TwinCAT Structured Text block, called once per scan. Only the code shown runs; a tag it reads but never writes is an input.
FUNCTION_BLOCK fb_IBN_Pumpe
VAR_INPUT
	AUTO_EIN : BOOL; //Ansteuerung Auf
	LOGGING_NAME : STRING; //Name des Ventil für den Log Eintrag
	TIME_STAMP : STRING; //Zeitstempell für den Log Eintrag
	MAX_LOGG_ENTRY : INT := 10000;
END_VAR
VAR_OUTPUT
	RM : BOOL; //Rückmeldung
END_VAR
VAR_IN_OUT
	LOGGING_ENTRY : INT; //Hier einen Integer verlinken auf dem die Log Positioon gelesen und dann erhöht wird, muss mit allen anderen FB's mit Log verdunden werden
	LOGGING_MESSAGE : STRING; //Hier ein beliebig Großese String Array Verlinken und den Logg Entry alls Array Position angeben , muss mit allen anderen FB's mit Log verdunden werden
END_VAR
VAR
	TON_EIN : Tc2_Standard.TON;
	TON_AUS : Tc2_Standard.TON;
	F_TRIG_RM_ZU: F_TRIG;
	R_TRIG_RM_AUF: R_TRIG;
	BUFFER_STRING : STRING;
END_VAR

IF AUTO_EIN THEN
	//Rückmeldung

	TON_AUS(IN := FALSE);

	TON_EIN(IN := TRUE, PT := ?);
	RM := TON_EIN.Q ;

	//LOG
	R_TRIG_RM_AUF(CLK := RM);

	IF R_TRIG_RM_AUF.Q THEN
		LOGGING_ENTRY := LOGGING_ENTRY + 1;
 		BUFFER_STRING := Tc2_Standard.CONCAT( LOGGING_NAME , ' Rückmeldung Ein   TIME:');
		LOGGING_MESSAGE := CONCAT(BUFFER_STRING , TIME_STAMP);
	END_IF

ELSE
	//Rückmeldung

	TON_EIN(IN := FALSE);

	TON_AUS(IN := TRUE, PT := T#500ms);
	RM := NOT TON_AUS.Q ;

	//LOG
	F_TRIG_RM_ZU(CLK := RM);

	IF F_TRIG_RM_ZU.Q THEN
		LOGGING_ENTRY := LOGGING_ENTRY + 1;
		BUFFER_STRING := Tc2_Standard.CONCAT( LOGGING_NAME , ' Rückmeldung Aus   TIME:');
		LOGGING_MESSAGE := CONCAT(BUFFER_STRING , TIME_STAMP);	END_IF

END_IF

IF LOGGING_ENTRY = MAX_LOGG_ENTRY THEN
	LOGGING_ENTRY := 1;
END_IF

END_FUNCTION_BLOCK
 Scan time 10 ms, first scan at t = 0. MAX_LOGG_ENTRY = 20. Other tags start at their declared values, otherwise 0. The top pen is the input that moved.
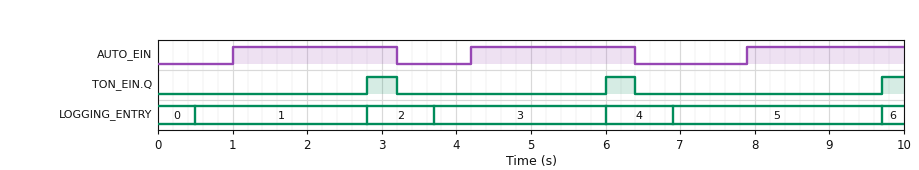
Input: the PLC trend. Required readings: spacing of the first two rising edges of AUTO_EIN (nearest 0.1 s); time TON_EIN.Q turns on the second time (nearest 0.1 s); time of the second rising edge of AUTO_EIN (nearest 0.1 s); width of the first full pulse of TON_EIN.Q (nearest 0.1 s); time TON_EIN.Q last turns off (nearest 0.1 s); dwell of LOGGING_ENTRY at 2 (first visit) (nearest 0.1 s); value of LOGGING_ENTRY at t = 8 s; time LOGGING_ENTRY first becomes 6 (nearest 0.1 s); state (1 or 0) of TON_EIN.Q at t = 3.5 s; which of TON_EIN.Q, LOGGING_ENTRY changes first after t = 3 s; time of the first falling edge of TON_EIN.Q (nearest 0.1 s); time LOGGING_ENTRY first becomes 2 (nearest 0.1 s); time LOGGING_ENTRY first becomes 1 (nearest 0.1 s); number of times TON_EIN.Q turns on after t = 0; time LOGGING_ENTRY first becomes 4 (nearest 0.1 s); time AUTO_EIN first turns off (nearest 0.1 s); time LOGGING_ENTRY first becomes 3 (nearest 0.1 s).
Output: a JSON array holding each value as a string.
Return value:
["3.2 s", "6.0 s", "4.2 s", "0.4 s", "6.4 s", "0.9 s", "5", "9.7 s", "0", "TON_EIN.Q", "3.2 s", "2.8 s", "0.5 s", "3", "6.0 s", "3.2 s", "3.7 s"]
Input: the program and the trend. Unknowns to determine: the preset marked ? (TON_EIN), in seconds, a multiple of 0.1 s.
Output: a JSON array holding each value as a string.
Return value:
["1.8 s"]
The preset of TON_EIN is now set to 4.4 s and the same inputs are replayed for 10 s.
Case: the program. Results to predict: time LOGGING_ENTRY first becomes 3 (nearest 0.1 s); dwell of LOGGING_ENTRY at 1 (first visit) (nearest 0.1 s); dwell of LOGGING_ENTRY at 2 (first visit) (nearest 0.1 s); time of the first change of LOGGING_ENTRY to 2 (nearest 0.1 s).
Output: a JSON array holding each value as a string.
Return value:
["6.9 s", "3.2 s", "3.2 s", "3.7 s"]
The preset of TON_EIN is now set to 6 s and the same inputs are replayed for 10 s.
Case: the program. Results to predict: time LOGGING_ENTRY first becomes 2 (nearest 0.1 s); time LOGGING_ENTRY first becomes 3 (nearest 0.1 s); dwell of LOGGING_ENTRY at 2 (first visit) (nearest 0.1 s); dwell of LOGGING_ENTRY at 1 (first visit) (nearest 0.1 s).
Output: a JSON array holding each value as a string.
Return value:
["3.7 s", "6.9 s", "3.2 s", "3.2 s"]
